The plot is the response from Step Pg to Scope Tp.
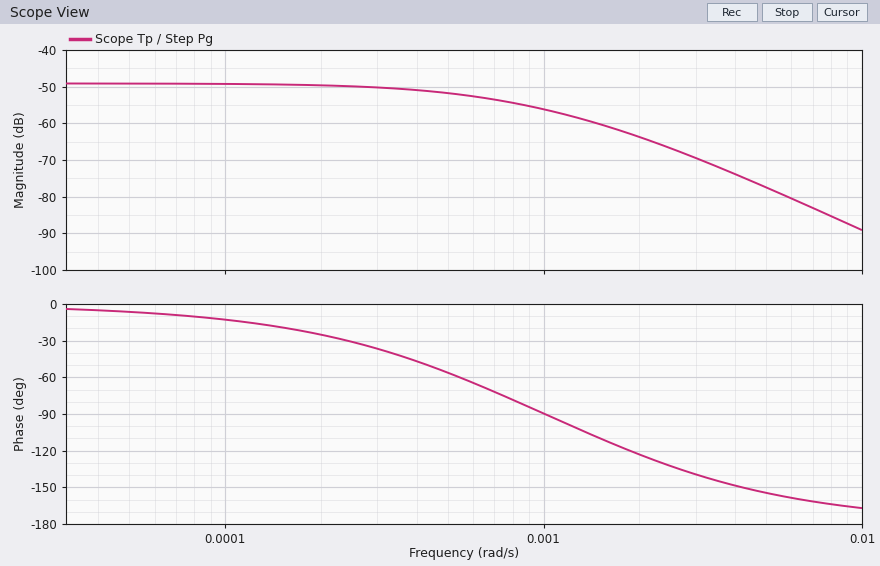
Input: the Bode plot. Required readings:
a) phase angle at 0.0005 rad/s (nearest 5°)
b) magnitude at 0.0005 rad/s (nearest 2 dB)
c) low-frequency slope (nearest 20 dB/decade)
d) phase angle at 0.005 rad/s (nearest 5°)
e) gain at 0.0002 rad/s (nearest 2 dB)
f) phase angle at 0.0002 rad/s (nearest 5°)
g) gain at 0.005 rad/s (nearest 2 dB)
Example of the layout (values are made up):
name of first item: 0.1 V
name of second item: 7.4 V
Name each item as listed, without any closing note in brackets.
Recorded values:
phase angle at 0.0005 rad/s: -55°
magnitude at 0.0005 rad/s: -52 dB
low-frequency slope: 0 dB/decade
phase angle at 0.005 rad/s: -155°
gain at 0.0002 rad/s: -50 dB
phase angle at 0.0002 rad/s: -25°
gain at 0.005 rad/s: -78 dB
